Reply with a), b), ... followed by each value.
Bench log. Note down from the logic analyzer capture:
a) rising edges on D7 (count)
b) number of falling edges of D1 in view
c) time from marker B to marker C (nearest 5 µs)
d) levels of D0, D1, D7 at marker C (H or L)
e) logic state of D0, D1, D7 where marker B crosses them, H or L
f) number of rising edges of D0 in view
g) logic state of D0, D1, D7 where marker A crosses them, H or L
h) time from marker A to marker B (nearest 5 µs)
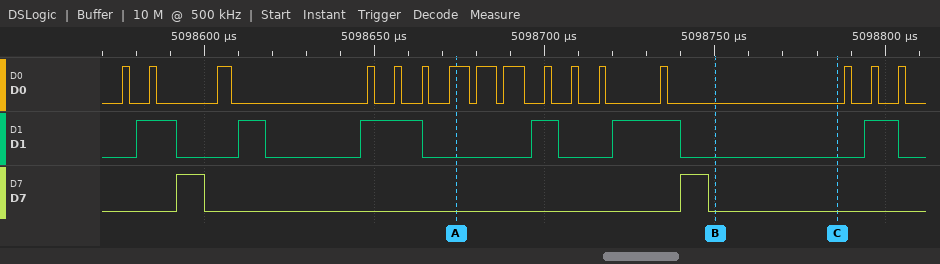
a) 2
b) 6
c) 35 µs
d) D0=L, D1=L, D7=L
e) D0=L, D1=L, D7=L
f) 16
g) D0=H, D1=L, D7=L
h) 75 µs
